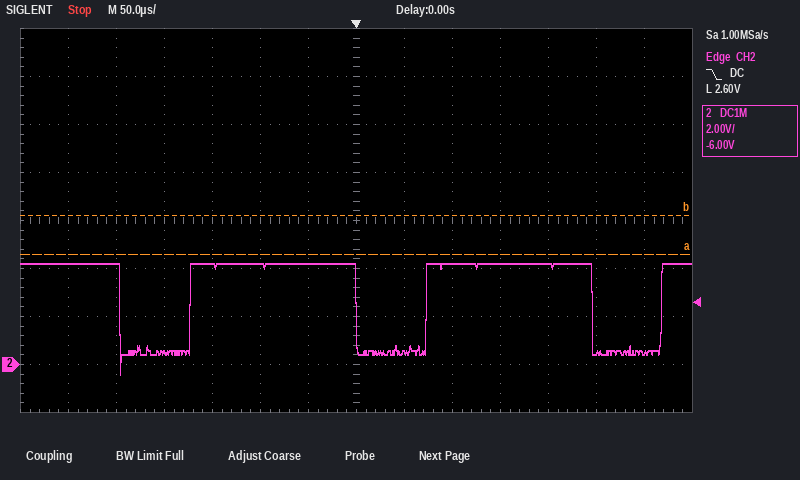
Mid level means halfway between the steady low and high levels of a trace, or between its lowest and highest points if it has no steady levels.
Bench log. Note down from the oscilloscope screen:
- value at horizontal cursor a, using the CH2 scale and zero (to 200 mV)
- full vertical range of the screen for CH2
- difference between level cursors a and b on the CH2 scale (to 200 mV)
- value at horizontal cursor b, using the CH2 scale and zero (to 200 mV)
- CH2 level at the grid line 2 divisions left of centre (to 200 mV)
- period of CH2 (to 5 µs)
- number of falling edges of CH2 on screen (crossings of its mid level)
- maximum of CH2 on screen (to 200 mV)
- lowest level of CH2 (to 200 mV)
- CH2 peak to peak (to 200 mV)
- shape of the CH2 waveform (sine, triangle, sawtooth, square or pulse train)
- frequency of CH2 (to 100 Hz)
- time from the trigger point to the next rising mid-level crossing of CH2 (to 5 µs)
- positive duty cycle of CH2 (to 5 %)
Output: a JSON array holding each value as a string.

["4.6 V", "16 V", "1.6 V", "6.2 V", "4.2 V", "245 µs", "3", "4.2 V", "-400 mV", "4.6 V", "pulse train", "4.1 kHz", "75 µs", "70 %"]
